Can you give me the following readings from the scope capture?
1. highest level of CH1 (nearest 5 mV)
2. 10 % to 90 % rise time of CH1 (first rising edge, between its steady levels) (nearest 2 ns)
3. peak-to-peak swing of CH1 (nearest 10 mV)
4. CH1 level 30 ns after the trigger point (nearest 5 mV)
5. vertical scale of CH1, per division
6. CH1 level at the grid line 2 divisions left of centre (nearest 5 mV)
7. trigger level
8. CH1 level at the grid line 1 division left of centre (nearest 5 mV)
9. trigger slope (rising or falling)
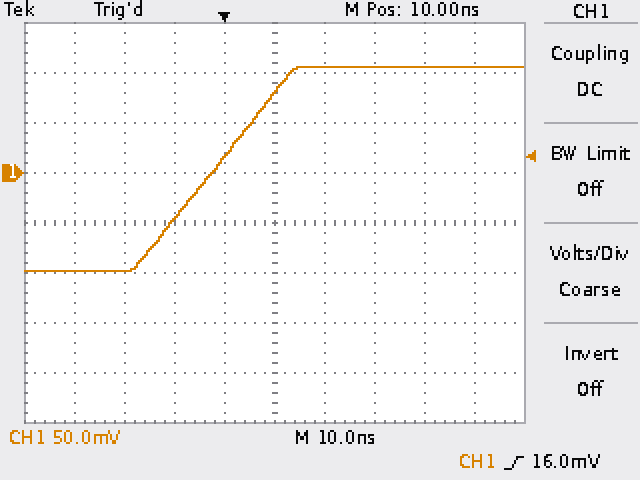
105 mV
26 ns
200 mV
105 mV
50 mV
-45 mV
16.0 mV
15 mV
rising
